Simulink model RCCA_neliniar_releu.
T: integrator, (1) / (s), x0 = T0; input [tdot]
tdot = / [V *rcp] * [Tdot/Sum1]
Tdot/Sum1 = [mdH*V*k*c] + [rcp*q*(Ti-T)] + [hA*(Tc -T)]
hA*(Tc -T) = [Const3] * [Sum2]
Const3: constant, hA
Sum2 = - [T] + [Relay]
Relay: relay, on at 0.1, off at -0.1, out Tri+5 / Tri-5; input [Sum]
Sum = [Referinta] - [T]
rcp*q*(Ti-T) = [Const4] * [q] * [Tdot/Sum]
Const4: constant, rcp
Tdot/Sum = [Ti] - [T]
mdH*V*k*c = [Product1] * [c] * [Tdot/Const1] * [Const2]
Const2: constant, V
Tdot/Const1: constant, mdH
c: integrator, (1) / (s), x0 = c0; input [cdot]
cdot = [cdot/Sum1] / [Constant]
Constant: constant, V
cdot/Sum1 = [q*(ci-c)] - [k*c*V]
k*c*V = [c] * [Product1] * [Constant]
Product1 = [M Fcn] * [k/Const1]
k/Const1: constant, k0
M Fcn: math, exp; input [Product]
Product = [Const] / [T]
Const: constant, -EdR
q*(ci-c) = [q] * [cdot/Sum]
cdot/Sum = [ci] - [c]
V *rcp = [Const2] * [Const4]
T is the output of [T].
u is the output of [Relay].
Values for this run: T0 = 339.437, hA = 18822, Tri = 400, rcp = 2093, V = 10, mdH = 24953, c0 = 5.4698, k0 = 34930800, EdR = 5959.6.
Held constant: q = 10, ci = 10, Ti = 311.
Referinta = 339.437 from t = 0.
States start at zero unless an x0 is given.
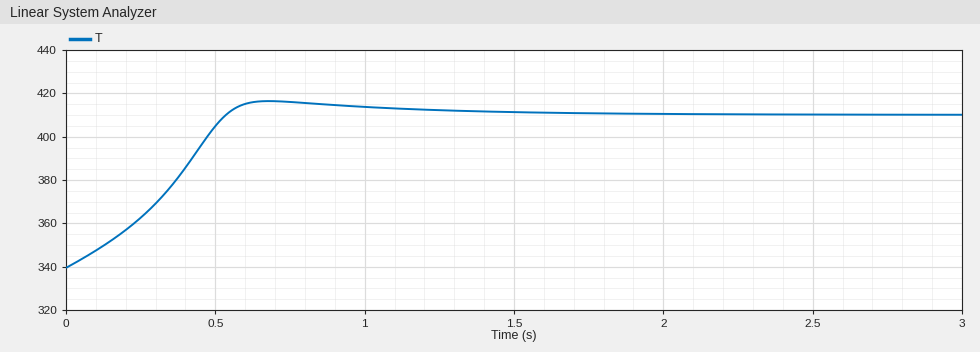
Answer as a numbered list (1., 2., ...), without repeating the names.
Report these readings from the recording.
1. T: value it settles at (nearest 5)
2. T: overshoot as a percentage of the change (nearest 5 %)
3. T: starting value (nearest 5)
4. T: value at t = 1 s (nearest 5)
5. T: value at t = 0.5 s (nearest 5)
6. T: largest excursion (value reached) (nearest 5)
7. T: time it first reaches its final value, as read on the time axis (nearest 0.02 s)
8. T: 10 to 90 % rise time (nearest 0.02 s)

1. 410
2. 10 %
3. 340
4. 415
5. 405
6. 415
7. 0.54 s
8. 0.40 s
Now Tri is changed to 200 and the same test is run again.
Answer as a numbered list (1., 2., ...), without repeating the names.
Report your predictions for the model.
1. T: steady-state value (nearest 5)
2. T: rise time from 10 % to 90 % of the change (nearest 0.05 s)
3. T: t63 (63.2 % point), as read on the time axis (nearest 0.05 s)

1. 260
2. 1.25 s
3. 0.60 s
